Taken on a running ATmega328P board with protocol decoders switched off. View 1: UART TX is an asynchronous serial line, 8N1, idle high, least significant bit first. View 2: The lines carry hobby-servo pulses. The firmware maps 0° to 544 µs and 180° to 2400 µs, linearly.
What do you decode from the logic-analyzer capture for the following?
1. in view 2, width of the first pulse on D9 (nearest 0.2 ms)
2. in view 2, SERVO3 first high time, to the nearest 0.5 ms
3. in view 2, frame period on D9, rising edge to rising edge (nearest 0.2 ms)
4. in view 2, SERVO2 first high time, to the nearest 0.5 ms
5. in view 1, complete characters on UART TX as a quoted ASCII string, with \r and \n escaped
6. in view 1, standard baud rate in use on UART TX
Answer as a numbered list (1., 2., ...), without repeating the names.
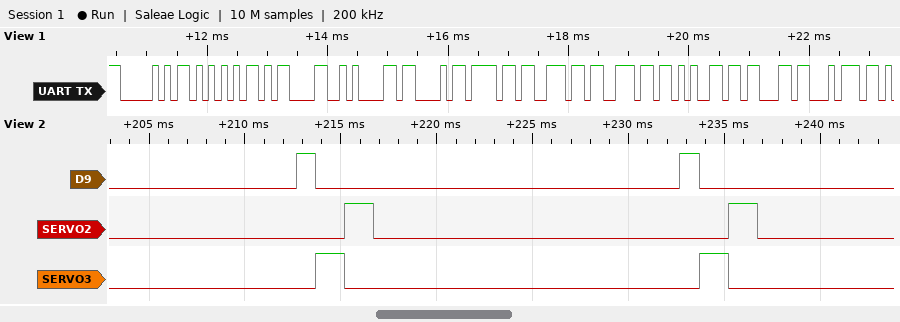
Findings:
1. 1.0 ms
2. 1.5 ms
3. 20.0 ms
4. 1.5 ms
5. "PU\r\nConnect"
6. 9600 baud
